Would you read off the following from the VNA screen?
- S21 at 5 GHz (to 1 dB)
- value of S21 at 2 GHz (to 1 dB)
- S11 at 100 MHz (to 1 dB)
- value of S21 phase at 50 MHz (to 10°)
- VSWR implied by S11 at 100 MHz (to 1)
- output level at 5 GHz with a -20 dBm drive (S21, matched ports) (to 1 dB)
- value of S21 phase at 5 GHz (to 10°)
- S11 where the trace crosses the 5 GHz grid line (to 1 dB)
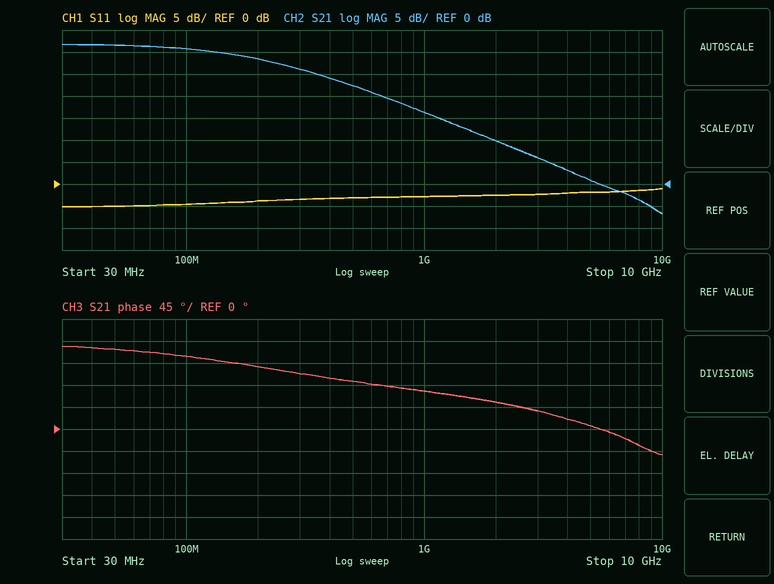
1 dB
10 dB
-5 dB
160°
4
-19 dBm
10°
-2 dB
